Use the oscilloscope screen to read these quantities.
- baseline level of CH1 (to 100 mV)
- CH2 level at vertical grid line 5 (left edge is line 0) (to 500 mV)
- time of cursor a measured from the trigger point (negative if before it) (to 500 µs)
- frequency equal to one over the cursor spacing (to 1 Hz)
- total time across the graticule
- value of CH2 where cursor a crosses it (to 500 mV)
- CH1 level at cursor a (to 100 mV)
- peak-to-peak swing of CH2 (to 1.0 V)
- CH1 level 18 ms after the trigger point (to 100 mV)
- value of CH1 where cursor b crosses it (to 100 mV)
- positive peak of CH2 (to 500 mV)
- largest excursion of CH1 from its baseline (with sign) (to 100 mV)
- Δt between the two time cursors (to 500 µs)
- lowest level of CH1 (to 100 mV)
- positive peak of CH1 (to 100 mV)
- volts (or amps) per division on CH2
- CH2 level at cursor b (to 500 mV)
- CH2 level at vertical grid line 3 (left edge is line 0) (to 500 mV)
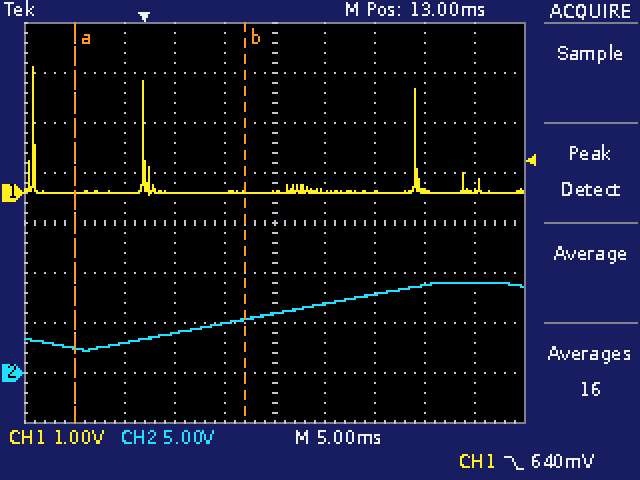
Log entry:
0.0 V
6.0 V
-7.0 ms
59 Hz
50 ms
2.5 V
0.0 V
7.0 V
0.0 V
0.0 V
9.0 V
+2.5 V
17.0 ms
0.0 V
2.5 V
5 V
5.5 V
4.0 V
